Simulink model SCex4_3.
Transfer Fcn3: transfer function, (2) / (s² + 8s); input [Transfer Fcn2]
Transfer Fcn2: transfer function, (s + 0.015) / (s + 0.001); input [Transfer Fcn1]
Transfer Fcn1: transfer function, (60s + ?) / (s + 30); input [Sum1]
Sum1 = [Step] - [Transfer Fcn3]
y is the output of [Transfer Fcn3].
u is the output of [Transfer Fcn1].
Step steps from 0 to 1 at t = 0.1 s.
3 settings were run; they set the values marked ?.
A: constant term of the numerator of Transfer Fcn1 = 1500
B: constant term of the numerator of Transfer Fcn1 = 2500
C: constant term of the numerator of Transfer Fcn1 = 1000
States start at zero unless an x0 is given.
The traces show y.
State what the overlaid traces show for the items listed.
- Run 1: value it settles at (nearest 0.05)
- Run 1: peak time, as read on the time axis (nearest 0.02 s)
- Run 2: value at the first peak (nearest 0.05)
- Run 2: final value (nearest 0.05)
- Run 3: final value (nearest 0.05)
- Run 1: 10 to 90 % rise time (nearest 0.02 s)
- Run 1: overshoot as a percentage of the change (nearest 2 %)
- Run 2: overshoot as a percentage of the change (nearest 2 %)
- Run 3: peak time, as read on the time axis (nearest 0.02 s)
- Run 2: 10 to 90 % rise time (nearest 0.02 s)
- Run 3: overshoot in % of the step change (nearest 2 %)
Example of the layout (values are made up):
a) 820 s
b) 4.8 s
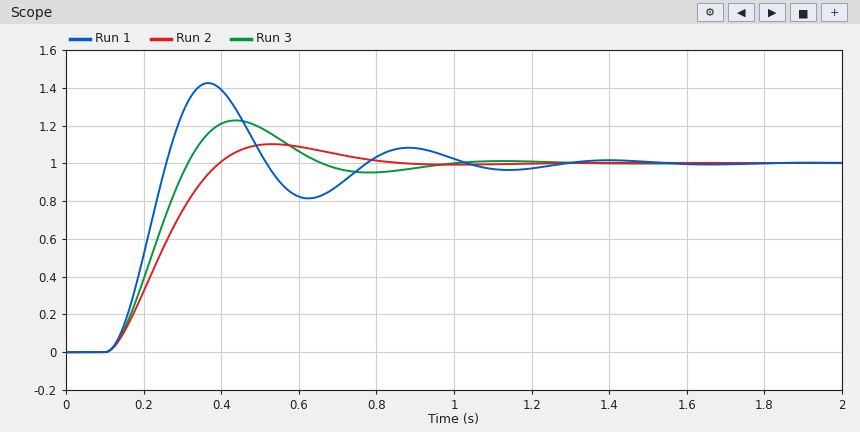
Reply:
a) 1.00
b) 0.36 s
c) 1.10
d) 1.00
e) 1.00
f) 0.10 s
g) 42 %
h) 10 %
i) 0.44 s
j) 0.20 s
k) 22 %
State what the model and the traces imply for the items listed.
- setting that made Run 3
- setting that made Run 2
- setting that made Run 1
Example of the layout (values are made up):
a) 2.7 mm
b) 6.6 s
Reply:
a) A
b) C
c) B
